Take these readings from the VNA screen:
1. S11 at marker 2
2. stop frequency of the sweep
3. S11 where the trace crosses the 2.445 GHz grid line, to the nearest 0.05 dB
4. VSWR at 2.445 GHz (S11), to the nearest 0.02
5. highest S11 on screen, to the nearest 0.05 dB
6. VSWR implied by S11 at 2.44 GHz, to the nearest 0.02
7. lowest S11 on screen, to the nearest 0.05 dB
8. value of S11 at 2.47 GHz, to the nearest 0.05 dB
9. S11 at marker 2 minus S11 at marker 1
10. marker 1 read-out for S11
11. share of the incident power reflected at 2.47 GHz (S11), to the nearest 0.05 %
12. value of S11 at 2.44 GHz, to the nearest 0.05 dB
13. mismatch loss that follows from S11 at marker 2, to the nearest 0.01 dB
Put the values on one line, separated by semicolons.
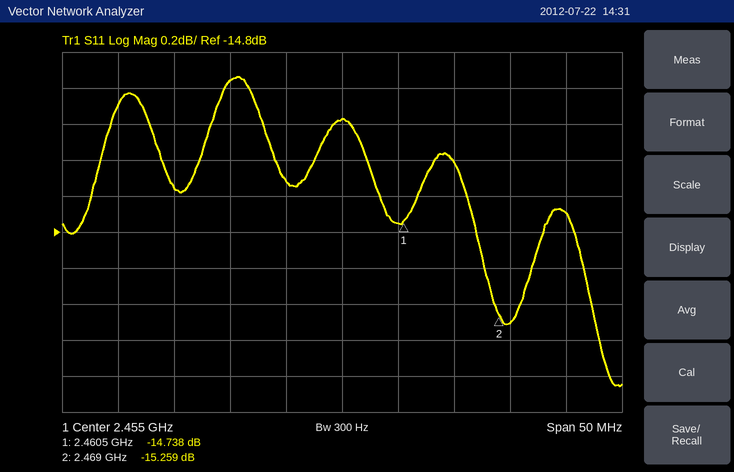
-15.259 dB; 2.48 GHz; -13.95 dB; 1.50; -13.95 dB; 1.46; -15.65 dB; -15.30 dB; -0.521 dB; -14.738 dB; 2.95 %; -14.55 dB; 0.13 dB
